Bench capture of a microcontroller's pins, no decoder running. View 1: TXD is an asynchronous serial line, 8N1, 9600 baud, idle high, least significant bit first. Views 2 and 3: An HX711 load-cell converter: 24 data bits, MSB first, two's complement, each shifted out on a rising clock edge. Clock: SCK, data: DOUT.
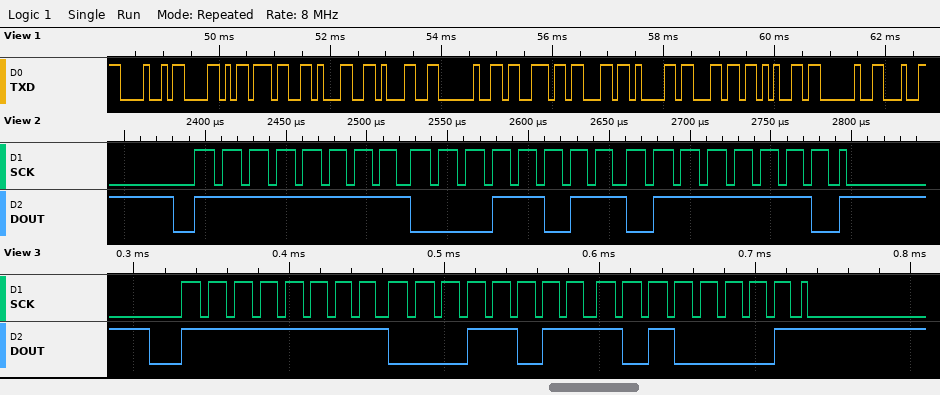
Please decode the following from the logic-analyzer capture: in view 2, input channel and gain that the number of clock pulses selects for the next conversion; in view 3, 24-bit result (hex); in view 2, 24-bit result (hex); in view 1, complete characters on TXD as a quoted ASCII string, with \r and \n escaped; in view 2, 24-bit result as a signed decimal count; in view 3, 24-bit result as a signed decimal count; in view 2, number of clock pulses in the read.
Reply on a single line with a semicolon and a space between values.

channel A, gain 128; 0xFF1BA1; 0xFF1B7E; "HX711 scale "; -58498; -58463; 25
